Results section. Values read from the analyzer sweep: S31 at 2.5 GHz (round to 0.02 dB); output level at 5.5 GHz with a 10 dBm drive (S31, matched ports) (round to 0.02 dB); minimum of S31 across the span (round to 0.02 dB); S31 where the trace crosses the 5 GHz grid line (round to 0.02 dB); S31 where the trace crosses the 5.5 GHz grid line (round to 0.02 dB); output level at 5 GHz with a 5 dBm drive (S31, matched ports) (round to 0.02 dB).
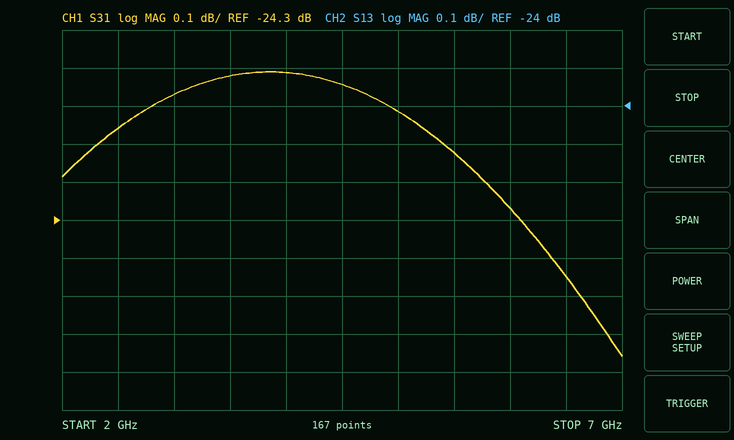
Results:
-24.06 dB
-14.12 dBm
-24.66 dB
-24.02 dB
-24.12 dB
-19.02 dBm
